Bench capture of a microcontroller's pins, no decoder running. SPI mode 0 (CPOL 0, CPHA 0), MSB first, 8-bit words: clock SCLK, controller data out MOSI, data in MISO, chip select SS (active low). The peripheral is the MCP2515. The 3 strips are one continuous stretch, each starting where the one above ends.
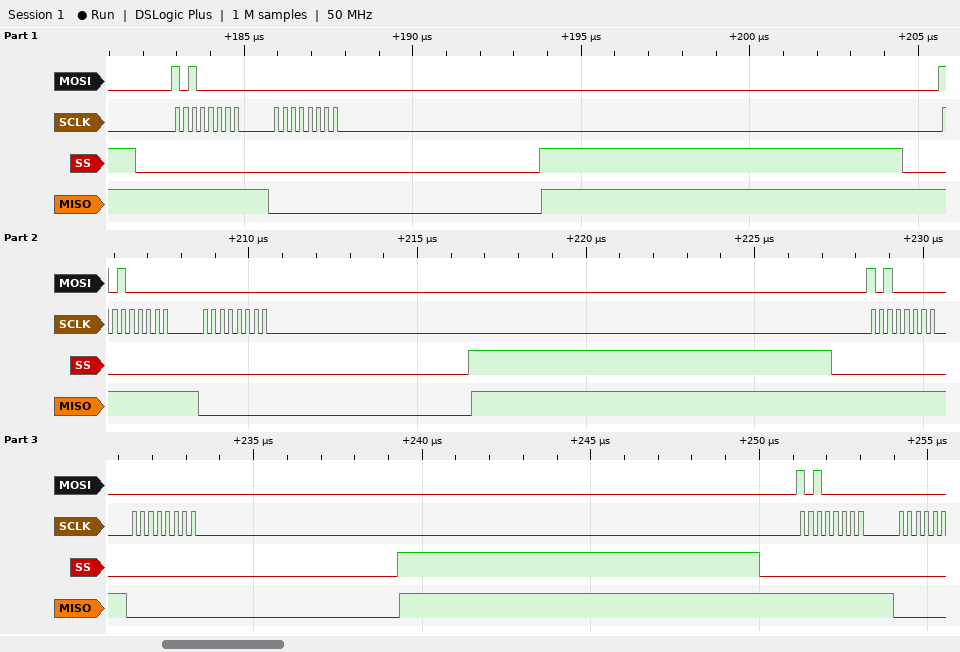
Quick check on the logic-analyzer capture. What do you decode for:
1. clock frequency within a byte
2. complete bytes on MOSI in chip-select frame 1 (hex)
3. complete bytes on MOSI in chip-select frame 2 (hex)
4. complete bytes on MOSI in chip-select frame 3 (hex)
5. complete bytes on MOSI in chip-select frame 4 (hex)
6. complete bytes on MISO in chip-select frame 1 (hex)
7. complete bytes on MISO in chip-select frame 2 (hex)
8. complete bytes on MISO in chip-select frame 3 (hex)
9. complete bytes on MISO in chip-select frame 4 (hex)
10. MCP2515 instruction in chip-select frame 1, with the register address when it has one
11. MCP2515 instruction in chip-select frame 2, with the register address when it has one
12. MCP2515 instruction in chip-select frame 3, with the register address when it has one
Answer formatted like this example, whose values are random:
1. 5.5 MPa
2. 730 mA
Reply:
1. 4 MHz
2. A0 00
3. A0 00
4. A0 00
5. A0
6. FF 00
7. FF 00
8. FF 00
9. FF
10. READ STATUS
11. READ STATUS
12. READ STATUS
